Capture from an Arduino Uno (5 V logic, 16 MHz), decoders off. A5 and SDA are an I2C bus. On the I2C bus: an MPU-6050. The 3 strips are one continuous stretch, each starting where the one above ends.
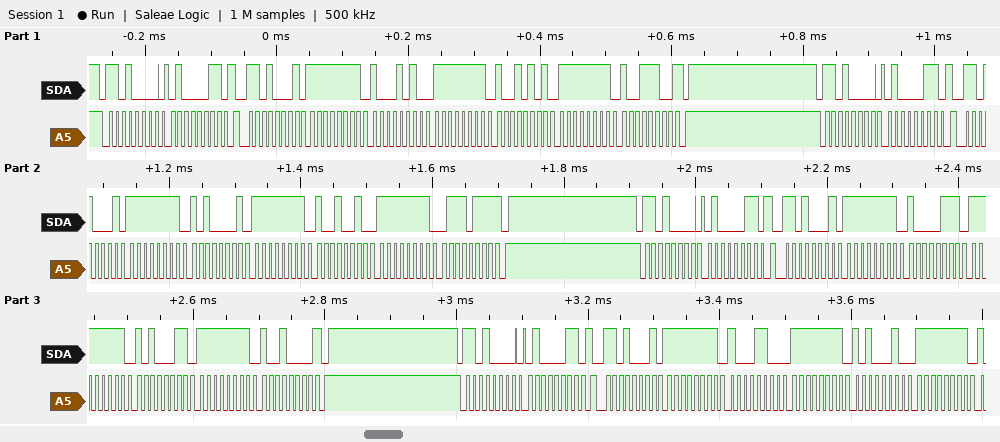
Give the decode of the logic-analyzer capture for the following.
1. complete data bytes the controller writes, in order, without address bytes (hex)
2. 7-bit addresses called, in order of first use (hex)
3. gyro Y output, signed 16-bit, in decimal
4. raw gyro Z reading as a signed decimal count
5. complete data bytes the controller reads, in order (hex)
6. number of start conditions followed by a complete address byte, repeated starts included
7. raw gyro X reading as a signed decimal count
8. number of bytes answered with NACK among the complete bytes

43 43 43 43
0x68
-107
-100
FF 8A FF 95 FF 9C FF A1 FF 92 FF 77 FF 87 FF A3 FF 90 FF 8C FF A2 FF
8
-118
3
